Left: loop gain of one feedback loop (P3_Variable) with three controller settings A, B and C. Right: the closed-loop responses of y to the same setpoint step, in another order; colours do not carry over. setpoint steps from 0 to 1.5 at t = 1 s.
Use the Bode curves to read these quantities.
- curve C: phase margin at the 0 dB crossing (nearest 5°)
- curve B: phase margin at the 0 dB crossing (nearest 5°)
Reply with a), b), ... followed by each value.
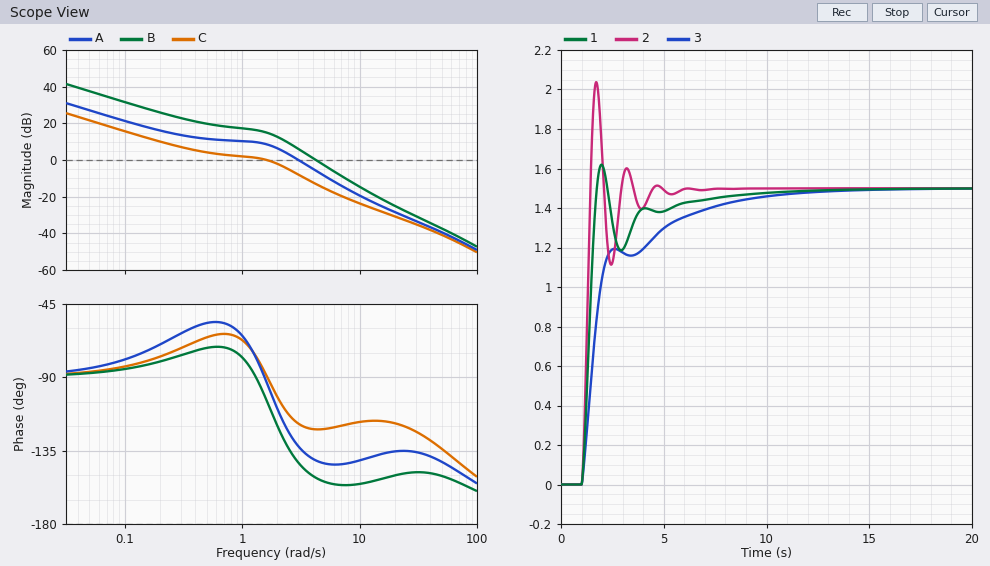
a) 90°
b) 30°
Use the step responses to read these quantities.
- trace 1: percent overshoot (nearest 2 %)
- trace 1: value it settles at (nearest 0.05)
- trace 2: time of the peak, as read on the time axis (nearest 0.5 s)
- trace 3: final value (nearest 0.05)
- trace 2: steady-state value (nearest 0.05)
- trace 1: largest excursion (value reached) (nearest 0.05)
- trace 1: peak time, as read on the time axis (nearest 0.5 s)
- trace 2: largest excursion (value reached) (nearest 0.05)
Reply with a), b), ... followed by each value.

a) 8 %
b) 1.50
c) 1.5 s
d) 1.50
e) 1.50
f) 1.60
g) 2.0 s
h) 2.05
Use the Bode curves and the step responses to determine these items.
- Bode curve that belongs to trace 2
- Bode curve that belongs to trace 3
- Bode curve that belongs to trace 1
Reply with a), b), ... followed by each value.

a) B
b) C
c) A
